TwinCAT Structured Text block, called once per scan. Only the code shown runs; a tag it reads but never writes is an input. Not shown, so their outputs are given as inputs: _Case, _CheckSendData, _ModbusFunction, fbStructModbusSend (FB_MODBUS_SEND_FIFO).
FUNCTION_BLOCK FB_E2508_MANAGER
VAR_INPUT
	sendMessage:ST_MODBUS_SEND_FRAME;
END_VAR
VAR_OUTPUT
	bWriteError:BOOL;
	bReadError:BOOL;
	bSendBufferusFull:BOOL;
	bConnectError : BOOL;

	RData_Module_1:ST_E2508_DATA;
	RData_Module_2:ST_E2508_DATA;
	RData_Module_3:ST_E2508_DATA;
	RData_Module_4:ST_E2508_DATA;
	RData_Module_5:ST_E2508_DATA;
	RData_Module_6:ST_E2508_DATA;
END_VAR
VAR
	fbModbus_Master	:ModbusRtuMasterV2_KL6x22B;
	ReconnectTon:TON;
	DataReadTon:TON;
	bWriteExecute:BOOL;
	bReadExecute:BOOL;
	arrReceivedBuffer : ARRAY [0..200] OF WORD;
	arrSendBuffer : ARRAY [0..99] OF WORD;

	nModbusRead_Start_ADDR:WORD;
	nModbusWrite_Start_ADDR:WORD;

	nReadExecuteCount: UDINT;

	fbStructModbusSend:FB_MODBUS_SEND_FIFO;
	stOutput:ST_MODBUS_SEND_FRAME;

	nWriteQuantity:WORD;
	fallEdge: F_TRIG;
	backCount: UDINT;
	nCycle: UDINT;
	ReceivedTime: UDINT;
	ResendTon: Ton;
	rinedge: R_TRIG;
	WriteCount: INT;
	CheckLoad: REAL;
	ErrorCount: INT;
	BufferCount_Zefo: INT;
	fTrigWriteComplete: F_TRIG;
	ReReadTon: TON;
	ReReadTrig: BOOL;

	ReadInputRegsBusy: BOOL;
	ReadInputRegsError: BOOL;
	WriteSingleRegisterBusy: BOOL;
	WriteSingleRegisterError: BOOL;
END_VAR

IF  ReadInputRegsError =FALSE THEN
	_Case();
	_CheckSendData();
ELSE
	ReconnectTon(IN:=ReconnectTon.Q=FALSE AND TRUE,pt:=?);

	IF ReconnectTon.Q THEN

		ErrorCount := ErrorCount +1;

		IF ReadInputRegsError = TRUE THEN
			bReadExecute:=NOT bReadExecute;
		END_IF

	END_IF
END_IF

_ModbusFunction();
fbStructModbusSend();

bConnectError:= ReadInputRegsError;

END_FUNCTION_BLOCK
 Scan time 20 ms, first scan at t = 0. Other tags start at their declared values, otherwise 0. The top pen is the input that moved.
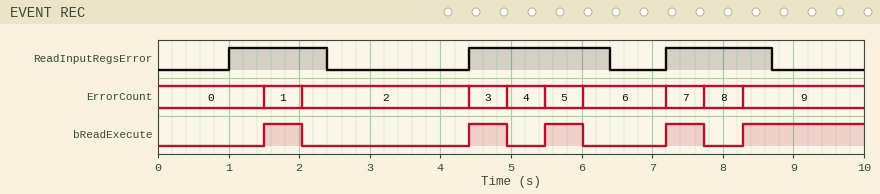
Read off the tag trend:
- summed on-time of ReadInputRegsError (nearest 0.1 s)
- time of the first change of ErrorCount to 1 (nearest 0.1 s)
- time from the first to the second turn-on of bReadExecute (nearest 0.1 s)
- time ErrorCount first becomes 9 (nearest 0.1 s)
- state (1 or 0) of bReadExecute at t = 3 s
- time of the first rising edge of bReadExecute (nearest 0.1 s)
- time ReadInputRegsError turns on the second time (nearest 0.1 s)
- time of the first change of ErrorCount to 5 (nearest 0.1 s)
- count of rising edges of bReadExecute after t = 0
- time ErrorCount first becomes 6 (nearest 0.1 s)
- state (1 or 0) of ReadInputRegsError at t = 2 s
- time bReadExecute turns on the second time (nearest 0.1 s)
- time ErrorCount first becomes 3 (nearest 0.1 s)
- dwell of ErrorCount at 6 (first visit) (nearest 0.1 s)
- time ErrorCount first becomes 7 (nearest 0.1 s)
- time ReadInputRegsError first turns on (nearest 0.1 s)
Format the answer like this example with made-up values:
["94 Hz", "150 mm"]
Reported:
["4.9 s", "1.5 s", "2.9 s", "8.3 s", "0", "1.5 s", "4.4 s", "5.5 s", "5", "6.0 s", "1", "4.4 s", "4.4 s", "1.2 s", "7.2 s", "1.0 s"]
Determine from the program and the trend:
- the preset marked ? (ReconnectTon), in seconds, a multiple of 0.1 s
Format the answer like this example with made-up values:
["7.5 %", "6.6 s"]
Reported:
["0.5 s"]
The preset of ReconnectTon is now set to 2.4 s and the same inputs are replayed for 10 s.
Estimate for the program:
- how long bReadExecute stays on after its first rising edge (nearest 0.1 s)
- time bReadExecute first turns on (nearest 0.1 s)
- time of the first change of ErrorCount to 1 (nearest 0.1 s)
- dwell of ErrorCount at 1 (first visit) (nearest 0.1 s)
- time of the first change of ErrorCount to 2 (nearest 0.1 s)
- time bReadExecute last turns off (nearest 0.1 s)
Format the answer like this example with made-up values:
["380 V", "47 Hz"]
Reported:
["2.8 s", "4.4 s", "4.4 s", "2.8 s", "7.2 s", "7.2 s"]
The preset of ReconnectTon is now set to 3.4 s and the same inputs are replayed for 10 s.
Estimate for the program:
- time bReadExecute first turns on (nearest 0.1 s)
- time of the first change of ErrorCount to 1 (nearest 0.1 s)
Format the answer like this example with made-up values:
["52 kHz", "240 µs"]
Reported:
["4.4 s", "4.4 s"]
